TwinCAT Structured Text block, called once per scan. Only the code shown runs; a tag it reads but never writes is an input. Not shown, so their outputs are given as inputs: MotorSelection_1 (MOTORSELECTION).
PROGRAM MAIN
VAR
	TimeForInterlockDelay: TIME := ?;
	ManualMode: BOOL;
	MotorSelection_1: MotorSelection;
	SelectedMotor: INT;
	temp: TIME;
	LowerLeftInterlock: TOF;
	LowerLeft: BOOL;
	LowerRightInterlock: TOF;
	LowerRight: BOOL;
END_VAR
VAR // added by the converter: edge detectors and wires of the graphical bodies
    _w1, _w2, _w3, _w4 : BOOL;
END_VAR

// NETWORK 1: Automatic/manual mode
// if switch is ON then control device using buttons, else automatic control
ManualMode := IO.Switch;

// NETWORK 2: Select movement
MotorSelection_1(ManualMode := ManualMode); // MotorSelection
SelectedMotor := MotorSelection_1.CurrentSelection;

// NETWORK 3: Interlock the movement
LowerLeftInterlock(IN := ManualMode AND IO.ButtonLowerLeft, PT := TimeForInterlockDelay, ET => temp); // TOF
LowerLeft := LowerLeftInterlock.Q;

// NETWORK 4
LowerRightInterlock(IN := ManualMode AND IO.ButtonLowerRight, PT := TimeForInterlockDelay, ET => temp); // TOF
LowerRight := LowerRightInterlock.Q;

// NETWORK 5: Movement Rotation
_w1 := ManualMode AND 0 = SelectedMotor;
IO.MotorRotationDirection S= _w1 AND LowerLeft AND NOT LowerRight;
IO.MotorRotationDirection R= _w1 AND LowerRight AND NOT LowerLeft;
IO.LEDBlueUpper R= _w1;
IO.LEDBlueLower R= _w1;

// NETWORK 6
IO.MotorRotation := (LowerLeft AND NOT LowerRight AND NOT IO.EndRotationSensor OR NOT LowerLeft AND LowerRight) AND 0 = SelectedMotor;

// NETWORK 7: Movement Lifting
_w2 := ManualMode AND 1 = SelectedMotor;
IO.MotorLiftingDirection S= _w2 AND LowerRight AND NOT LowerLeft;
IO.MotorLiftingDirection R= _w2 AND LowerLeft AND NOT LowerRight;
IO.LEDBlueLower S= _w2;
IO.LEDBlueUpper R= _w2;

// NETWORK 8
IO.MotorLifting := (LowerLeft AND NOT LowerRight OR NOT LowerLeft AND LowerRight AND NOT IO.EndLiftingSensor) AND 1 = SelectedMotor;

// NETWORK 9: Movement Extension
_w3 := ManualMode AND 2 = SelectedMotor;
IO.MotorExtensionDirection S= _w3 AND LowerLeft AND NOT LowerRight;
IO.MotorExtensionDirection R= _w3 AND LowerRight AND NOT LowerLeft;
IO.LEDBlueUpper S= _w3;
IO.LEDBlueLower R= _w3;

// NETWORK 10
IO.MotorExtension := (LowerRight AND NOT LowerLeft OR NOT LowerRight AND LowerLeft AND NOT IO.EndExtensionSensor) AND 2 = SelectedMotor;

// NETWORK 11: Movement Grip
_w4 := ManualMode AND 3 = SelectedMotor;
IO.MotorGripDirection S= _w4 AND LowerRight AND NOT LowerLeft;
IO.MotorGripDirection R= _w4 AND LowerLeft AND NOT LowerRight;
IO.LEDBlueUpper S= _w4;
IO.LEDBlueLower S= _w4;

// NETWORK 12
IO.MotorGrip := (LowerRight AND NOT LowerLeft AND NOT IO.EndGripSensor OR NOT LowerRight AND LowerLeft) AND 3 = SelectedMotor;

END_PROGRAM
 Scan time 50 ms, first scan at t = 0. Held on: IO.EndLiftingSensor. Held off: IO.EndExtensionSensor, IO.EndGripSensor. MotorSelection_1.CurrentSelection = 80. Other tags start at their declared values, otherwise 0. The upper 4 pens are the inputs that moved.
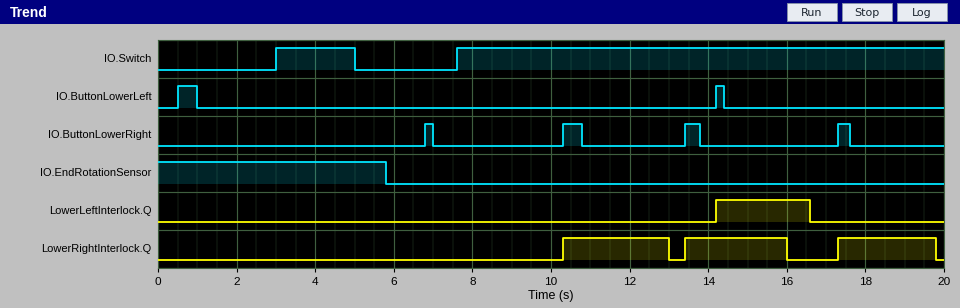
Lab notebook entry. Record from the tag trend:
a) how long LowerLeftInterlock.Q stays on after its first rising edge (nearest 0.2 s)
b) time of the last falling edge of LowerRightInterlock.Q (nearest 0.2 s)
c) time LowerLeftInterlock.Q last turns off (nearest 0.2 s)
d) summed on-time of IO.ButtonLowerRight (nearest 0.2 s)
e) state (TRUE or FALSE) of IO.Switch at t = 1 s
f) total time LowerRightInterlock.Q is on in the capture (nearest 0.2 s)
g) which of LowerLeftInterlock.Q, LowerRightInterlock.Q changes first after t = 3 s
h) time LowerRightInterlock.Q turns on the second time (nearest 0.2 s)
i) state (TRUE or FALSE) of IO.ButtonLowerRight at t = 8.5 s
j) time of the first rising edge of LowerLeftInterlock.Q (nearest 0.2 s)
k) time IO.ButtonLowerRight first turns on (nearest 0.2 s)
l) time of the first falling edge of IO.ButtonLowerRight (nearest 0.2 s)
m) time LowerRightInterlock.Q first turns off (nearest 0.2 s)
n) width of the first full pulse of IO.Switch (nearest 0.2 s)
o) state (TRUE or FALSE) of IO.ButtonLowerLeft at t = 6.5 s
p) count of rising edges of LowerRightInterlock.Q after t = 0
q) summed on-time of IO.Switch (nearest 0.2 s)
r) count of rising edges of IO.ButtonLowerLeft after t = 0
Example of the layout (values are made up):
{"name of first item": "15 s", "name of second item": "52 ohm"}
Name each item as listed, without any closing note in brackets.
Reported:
{"how long LowerLeftInterlock.Q stays on after its first rising edge": "2.4 s", "time of the last falling edge of LowerRightInterlock.Q": "19.8 s", "time LowerLeftInterlock.Q last turns off": "16.6 s", "summed on-time of IO.ButtonLowerRight": "1.4 s", "state (TRUE or FALSE) of IO.Switch at t = 1 s": "FALSE", "total time LowerRightInterlock.Q is on in the capture": "7.8 s", "which of LowerLeftInterlock.Q, LowerRightInterlock.Q changes first after t = 3 s": "LowerRightInterlock.Q", "time LowerRightInterlock.Q turns on the second time": "13.4 s", "state (TRUE or FALSE) of IO.ButtonLowerRight at t = 8.5 s": "FALSE", "time of the first rising edge of LowerLeftInterlock.Q": "14.2 s", "time IO.ButtonLowerRight first turns on": "6.8 s", "time of the first falling edge of IO.ButtonLowerRight": "7.0 s", "time LowerRightInterlock.Q first turns off": "13.0 s", "width of the first full pulse of IO.Switch": "2.0 s", "state (TRUE or FALSE) of IO.ButtonLowerLeft at t = 6.5 s": "FALSE", "count of rising edges of LowerRightInterlock.Q after t = 0": "3", "summed on-time of IO.Switch": "14.4 s", "count of rising edges of IO.ButtonLowerLeft after t = 0": "2"}
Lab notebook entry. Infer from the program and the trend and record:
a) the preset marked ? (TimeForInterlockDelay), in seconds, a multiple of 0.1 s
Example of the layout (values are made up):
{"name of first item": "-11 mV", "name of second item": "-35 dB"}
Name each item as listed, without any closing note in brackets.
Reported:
{"the preset marked ? (TimeForInterlockDelay), in seconds, a multiple of 0.1 s": "2.2 s"}
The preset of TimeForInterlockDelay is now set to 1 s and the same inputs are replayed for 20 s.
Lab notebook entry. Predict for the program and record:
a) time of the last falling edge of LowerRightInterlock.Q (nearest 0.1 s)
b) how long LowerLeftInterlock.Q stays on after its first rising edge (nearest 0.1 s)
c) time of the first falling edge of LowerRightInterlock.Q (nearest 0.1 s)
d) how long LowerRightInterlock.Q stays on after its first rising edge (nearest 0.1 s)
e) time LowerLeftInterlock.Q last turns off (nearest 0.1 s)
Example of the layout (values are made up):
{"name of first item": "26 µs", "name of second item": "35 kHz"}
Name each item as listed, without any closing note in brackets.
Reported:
{"time of the last falling edge of LowerRightInterlock.Q": "18.6 s", "how long LowerLeftInterlock.Q stays on after its first rising edge": "1.2 s", "time of the first falling edge of LowerRightInterlock.Q": "11.8 s", "how long LowerRightInterlock.Q stays on after its first rising edge": "1.5 s", "time LowerLeftInterlock.Q last turns off": "15.4 s"}
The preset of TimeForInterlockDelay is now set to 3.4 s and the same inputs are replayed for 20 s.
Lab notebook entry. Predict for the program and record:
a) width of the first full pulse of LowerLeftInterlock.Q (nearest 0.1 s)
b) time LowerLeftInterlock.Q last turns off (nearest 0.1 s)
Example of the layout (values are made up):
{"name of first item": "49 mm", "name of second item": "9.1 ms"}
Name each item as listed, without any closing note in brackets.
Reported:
{"width of the first full pulse of LowerLeftInterlock.Q": "3.6 s", "time LowerLeftInterlock.Q last turns off": "17.8 s"}
